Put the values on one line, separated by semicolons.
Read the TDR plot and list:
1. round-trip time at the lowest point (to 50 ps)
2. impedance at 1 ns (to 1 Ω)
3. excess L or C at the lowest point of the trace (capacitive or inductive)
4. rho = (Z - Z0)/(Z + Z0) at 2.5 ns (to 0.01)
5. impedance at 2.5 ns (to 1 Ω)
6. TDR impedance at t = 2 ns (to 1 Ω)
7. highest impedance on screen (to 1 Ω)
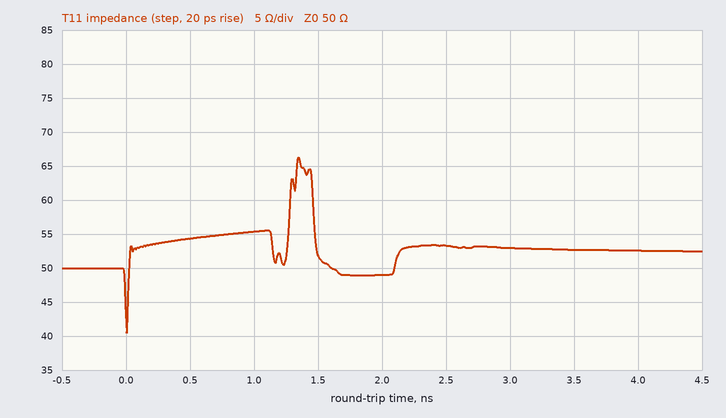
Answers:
0 ps; 55 Ω; capacitive; +0.03; 53 Ω; 49 Ω; 66 Ω
